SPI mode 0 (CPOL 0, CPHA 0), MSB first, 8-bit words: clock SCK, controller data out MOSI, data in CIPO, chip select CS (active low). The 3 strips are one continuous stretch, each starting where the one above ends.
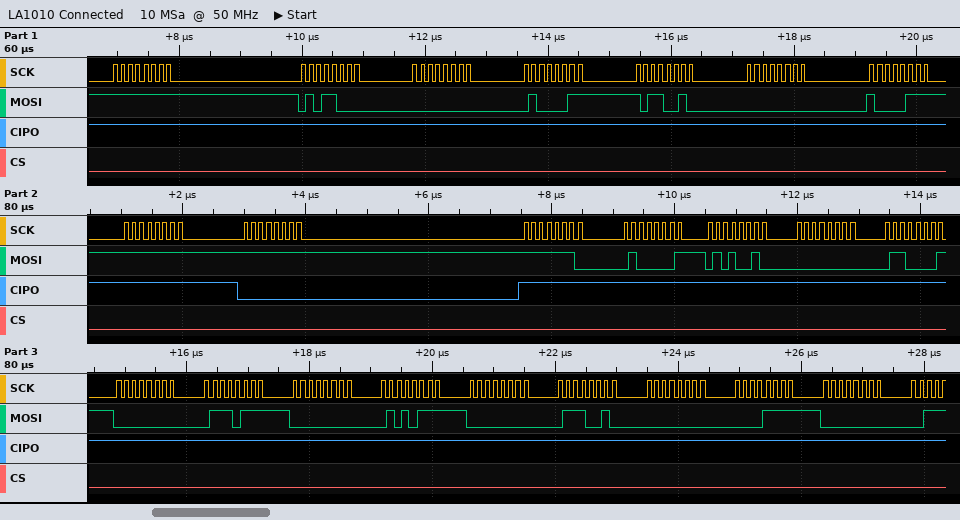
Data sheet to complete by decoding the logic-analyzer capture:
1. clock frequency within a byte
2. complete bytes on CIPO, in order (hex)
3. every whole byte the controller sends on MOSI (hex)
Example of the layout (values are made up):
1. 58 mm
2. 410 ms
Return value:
1. 8 MHz
2. 0xFF 0xFF 0xFF 0xFF 0xFF 0xFF 0xFF 0xFF 0x00 0xFF 0xFF 0xFF 0xFF 0xFF 0xFF 0xFF 0xFF 0xFF 0xFF 0xFF 0xFF 0xFF 0xFF
3. 0xFF 0x58 0x00 0x43 0xB2 0x00 0x87 0xFF 0xFF 0xFE 0x41 0x52 0x00 0x61 0x00 0x77 0x00 0x57 0x00 0x72 0x00 0x0F 0x00
